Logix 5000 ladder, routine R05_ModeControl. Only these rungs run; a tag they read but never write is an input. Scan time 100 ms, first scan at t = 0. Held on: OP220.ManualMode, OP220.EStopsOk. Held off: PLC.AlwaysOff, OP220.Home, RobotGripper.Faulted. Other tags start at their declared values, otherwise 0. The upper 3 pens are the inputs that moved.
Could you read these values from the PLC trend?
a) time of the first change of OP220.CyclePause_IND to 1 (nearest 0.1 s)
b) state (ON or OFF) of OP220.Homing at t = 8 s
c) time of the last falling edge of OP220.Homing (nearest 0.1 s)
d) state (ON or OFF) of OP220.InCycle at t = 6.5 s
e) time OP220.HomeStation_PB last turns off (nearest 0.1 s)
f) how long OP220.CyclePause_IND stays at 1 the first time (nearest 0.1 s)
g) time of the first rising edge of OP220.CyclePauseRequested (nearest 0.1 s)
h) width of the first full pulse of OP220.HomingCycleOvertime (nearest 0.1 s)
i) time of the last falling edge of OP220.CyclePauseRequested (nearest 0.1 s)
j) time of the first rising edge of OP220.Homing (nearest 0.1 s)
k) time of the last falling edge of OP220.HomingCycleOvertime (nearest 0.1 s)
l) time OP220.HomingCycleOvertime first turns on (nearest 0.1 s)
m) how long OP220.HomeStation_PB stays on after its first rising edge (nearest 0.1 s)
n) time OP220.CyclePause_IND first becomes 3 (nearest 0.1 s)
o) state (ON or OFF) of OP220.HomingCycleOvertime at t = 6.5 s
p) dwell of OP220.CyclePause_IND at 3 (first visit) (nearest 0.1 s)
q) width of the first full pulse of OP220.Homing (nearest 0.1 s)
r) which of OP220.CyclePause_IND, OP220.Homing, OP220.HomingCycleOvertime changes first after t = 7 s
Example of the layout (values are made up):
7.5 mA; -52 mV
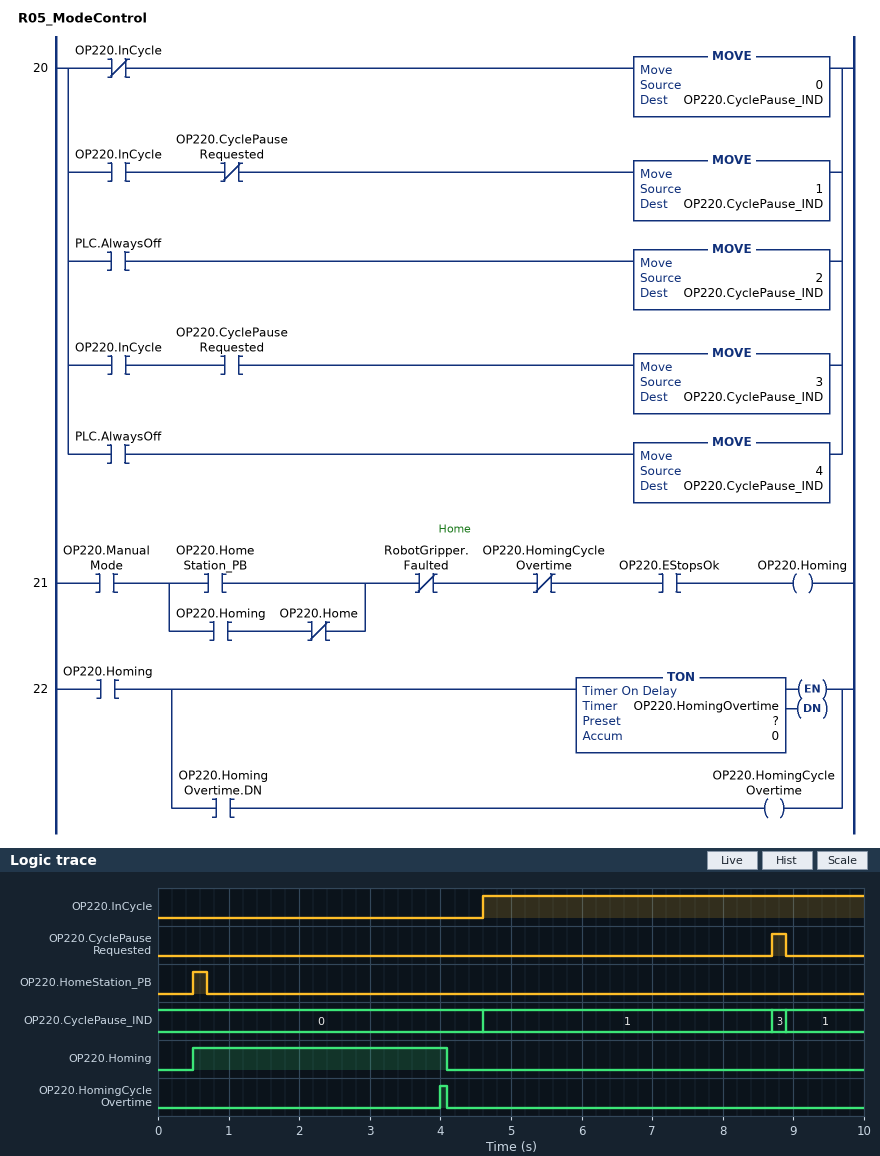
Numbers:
4.6 s; OFF; 4.1 s; ON; 0.7 s; 4.1 s; 8.7 s; 0.1 s; 8.9 s; 0.5 s; 4.1 s; 4.0 s; 0.2 s; 8.7 s; OFF; 0.2 s; 3.6 s; OP220.CyclePause_IND
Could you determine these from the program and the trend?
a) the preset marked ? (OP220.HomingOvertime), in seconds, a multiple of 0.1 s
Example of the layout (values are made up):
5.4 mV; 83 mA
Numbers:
3.5 s
